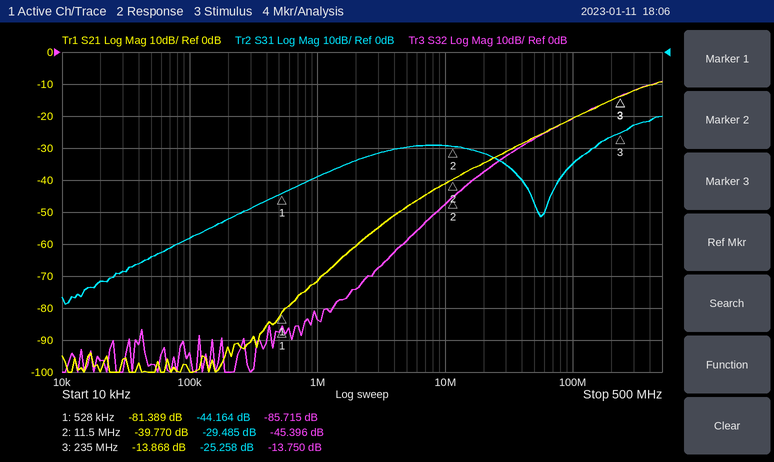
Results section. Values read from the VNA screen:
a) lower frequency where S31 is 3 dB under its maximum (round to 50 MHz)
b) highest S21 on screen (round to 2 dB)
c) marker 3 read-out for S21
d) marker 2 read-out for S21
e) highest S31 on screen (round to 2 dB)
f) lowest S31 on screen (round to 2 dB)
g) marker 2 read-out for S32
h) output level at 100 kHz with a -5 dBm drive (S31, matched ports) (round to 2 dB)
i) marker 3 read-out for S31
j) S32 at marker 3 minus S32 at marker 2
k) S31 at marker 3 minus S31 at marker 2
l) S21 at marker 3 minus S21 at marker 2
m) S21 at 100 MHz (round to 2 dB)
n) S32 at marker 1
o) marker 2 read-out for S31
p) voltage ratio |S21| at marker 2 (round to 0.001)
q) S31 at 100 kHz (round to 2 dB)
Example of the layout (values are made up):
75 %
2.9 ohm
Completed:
300 MHz
-10 dB
-13.868 dB
-39.770 dB
-20 dB
-78 dB
-45.396 dB
-64 dBm
-25.258 dB
31.646 dB
4.227 dB
25.902 dB
-20 dB
-85.715 dB
-29.485 dB
0.010
-58 dB
